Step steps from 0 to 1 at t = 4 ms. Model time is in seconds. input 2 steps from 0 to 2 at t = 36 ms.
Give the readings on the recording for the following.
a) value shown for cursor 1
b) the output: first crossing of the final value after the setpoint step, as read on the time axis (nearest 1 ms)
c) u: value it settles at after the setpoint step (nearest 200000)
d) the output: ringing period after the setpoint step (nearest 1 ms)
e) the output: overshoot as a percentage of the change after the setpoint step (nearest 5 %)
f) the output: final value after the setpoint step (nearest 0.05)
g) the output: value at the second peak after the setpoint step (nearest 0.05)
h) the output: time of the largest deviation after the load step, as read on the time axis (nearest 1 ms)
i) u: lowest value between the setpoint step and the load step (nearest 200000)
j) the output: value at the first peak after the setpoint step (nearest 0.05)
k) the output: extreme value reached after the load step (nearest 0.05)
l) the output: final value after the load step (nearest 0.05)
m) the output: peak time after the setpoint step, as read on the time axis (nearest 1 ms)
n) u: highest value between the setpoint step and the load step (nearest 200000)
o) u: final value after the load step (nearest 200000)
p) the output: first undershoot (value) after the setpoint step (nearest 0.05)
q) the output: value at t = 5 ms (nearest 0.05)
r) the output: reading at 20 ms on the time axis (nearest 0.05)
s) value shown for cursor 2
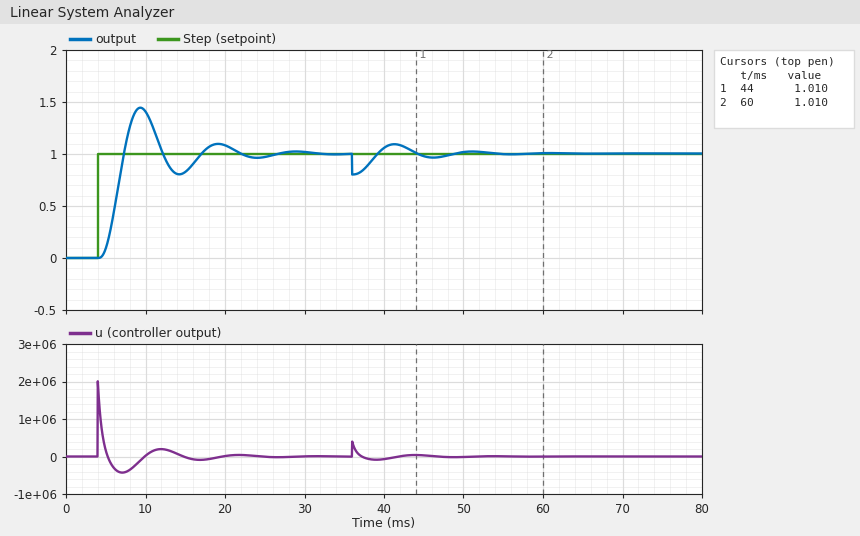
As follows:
1.010
7 ms
0
10 ms
45 %
1.00
1.10
36 ms
-400000
1.45
0.80
1.00
9 ms
2000000
0
0.80
0.10
1.10
1.010
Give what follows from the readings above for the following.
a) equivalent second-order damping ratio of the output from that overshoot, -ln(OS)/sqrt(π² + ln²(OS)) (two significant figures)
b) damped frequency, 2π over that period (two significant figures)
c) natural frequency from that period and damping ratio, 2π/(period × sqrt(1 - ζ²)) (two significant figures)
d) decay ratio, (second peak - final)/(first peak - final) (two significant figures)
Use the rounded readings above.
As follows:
0.25
0.63 rad/ms
0.65 rad/ms
0.22
